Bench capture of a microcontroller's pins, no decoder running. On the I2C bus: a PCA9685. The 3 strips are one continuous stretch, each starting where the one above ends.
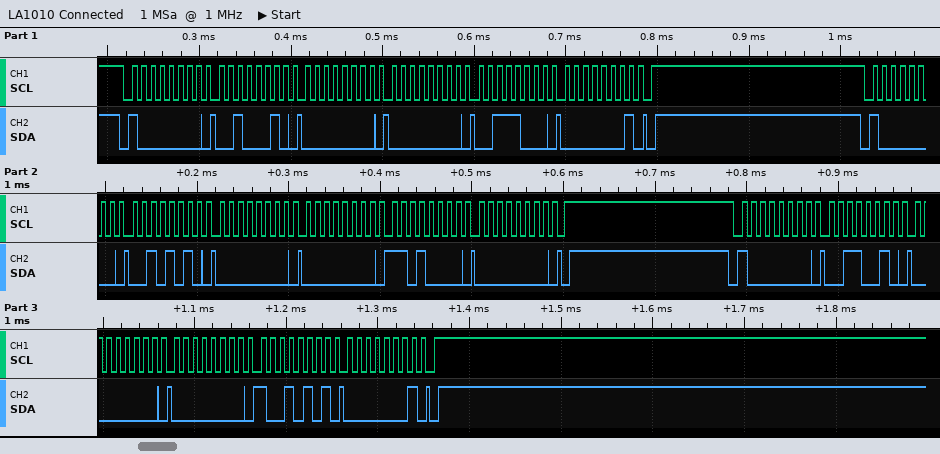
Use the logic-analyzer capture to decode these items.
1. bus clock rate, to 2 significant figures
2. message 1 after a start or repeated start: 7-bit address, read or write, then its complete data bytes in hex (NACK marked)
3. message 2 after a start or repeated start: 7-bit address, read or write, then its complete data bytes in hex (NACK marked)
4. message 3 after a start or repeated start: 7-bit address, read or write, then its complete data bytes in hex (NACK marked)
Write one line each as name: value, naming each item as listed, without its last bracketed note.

bus clock rate, to 2 significant figures: 100 kHz
message 1 after a start or repeated start: 7-bit address, read or write, then its complete data bytes in hex: 0x40 write: 22 00 00 38 01
message 2 after a start or repeated start: 7-bit address, read or write, then its complete data bytes in hex: 0x40 write: 2A 00 00 D0 00
message 3 after a start or repeated start: 7-bit address, read or write, then its complete data bytes in hex: 0x40 write: 32 00 00 95 01
